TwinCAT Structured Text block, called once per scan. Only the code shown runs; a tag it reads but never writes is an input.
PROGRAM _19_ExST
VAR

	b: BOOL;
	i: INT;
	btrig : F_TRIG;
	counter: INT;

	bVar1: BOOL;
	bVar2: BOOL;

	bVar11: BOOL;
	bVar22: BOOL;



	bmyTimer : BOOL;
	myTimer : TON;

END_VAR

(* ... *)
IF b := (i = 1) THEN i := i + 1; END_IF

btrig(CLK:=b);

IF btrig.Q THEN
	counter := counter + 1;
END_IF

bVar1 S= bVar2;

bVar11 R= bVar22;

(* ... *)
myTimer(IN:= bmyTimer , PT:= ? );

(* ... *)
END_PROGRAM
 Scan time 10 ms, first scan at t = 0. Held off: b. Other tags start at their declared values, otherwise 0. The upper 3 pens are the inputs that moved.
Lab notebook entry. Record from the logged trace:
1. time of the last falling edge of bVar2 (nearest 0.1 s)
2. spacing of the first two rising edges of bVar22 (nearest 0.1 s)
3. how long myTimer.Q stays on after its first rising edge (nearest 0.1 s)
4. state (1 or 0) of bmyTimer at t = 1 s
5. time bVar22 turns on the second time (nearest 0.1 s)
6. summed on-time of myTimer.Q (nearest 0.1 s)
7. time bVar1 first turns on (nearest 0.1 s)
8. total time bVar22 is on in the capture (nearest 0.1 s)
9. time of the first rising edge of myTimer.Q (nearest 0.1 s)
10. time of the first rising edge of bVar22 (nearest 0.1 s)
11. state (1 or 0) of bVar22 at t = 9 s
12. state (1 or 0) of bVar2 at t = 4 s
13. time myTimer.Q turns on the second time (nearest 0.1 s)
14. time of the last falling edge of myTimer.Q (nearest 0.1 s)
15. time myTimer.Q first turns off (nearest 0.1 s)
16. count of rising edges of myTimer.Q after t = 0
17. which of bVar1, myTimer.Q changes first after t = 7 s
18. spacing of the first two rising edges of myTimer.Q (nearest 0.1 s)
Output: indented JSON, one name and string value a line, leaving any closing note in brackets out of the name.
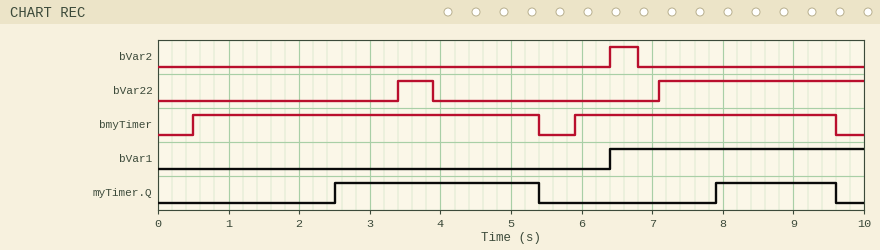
{
  "time of the last falling edge of bVar2": "6.8 s",
  "spacing of the first two rising edges of bVar22": "3.7 s",
  "how long myTimer.Q stays on after its first rising edge": "2.9 s",
  "state (1 or 0) of bmyTimer at t = 1 s": "1",
  "time bVar22 turns on the second time": "7.1 s",
  "summed on-time of myTimer.Q": "4.6 s",
  "time bVar1 first turns on": "6.4 s",
  "total time bVar22 is on in the capture": "3.4 s",
  "time of the first rising edge of myTimer.Q": "2.5 s",
  "time of the first rising edge of bVar22": "3.4 s",
  "state (1 or 0) of bVar22 at t = 9 s": "1",
  "state (1 or 0) of bVar2 at t = 4 s": "0",
  "time myTimer.Q turns on the second time": "7.9 s",
  "time of the last falling edge of myTimer.Q": "9.6 s",
  "time myTimer.Q first turns off": "5.4 s",
  "count of rising edges of myTimer.Q after t = 0": "2",
  "which of bVar1, myTimer.Q changes first after t = 7 s": "myTimer.Q",
  "spacing of the first two rising edges of myTimer.Q": "5.4 s"
}
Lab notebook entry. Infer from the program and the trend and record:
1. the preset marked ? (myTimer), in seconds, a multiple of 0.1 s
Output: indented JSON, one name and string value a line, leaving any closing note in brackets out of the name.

{
  "the preset marked ? (myTimer), in seconds, a multiple of 0.1 s": "2.0 s"
}
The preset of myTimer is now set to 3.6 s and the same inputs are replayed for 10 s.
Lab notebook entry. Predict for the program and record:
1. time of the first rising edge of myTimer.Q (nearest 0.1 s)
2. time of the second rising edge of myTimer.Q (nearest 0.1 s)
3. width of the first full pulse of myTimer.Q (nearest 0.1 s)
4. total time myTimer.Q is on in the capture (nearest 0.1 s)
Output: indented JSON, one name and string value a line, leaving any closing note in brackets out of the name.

{
  "time of the first rising edge of myTimer.Q": "4.1 s",
  "time of the second rising edge of myTimer.Q": "9.5 s",
  "width of the first full pulse of myTimer.Q": "1.3 s",
  "total time myTimer.Q is on in the capture": "1.4 s"
}
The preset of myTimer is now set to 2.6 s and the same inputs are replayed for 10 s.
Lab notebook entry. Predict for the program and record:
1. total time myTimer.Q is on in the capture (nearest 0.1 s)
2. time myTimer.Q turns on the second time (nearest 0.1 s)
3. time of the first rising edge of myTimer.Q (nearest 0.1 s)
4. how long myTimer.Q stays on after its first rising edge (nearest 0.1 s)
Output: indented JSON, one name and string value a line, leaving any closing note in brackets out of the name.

{
  "total time myTimer.Q is on in the capture": "3.4 s",
  "time myTimer.Q turns on the second time": "8.5 s",
  "time of the first rising edge of myTimer.Q": "3.1 s",
  "how long myTimer.Q stays on after its first rising edge": "2.3 s"
}
